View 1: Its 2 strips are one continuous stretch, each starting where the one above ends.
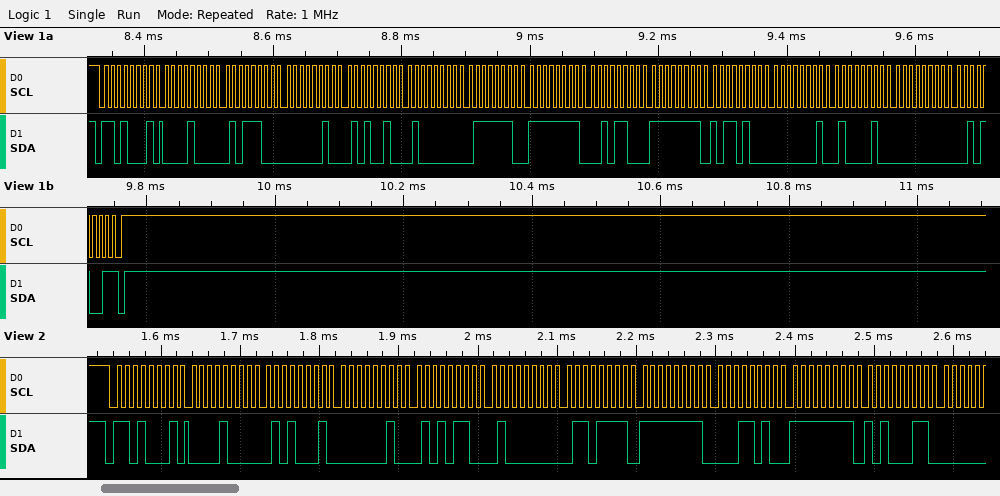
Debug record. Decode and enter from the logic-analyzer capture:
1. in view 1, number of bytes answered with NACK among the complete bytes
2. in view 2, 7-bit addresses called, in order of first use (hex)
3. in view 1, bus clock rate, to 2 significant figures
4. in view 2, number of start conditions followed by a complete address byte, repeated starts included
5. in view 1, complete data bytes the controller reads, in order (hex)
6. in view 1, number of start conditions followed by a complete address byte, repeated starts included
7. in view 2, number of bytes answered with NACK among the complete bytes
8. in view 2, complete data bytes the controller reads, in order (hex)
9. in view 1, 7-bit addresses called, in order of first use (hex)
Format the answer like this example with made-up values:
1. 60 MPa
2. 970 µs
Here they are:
1. 1
2. 0x68
3. 100 kHz
4. 1
5. 08 5C 02 52 40 7E FF 2C FF B4 01 42 00 29
6. 1
7. 0
8. 08 51 02 56 40 6F FF 1A FF A3
9. 0x68
